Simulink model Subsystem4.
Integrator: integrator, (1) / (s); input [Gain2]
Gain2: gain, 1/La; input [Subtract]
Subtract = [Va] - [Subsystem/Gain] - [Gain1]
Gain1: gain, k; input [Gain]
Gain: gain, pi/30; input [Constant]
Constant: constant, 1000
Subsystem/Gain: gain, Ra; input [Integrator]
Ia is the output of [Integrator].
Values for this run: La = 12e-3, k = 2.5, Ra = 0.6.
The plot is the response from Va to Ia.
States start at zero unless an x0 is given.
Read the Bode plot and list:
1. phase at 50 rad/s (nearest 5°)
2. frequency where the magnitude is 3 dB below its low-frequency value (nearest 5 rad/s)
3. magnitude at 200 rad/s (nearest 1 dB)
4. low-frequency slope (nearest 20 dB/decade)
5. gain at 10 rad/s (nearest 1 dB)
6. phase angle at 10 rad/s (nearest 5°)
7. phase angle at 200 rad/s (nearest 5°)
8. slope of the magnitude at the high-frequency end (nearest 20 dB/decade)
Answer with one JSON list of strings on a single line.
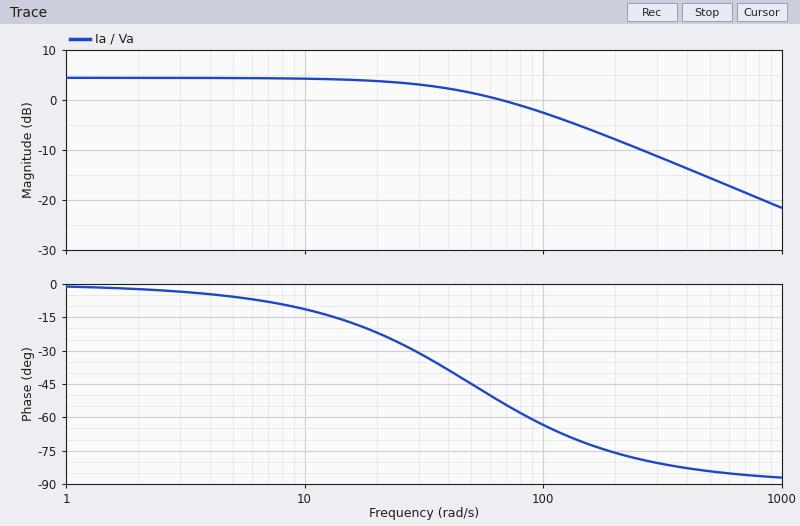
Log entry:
["-45°", "50 rad/s", "-8 dB", "0 dB/decade", "4 dB", "-10°", "-75°", "-20 dB/decade"]
